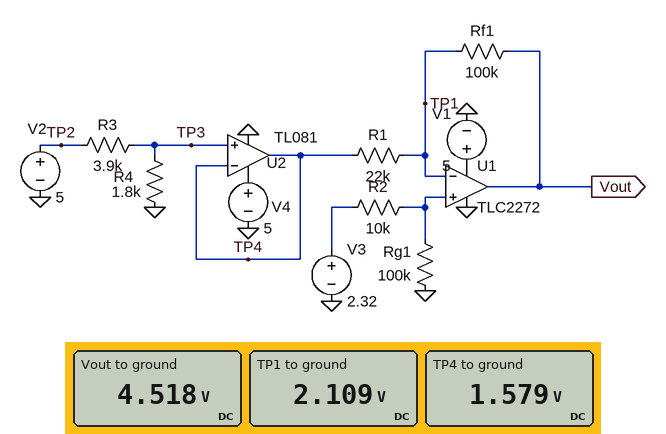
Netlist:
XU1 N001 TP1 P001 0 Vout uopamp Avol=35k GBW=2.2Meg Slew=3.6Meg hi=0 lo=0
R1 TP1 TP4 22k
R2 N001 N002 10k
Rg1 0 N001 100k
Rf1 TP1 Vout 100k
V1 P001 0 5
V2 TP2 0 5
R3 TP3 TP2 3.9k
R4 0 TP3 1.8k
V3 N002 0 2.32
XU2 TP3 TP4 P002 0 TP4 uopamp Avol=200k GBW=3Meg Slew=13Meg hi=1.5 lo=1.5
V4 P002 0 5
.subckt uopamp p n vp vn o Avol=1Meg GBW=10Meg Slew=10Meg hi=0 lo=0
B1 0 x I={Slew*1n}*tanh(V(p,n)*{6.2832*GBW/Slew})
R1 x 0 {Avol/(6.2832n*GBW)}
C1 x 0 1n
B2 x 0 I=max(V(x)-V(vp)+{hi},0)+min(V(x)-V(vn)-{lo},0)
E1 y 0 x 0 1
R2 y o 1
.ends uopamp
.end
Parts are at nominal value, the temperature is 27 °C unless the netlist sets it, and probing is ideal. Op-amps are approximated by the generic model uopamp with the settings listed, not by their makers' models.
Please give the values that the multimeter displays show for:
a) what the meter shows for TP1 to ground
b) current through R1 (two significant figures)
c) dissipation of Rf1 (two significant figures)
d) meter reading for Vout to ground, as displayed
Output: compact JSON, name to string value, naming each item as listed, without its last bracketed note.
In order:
{"what the meter shows for TP1 to ground": "2.109 V", "current through R1": "24 µA", "dissipation of Rf1": "58 µW", "meter reading for Vout to ground, as displayed": "4.518 V"}
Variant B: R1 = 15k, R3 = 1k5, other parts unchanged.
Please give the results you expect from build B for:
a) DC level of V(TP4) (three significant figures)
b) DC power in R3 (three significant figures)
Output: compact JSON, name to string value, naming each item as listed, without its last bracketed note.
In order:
{"DC level of V(TP4)": "2.73 V", "DC power in R3": "3.44 mW"}
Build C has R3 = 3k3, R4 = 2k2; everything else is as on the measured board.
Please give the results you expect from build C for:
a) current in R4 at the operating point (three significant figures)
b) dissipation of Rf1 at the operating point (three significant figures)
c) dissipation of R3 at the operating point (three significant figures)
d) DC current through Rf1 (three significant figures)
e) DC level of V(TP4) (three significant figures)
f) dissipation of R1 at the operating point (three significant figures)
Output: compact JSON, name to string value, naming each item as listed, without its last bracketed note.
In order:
{"current in R4 at the operating point": "909 µA", "dissipation of Rf1 at the operating point": "2.46 µW", "dissipation of R3 at the operating point": "2.73 mW", "DC current through Rf1": "4.96 µA", "DC level of V(TP4)": "2.00 V", "dissipation of R1 at the operating point": "540 nW"}
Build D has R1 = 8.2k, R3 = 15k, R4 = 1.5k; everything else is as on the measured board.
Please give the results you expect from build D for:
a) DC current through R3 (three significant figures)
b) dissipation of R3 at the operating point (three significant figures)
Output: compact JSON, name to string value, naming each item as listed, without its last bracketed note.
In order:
{"DC current through R3": "303 µA", "dissipation of R3 at the operating point": "1.38 mW"}
